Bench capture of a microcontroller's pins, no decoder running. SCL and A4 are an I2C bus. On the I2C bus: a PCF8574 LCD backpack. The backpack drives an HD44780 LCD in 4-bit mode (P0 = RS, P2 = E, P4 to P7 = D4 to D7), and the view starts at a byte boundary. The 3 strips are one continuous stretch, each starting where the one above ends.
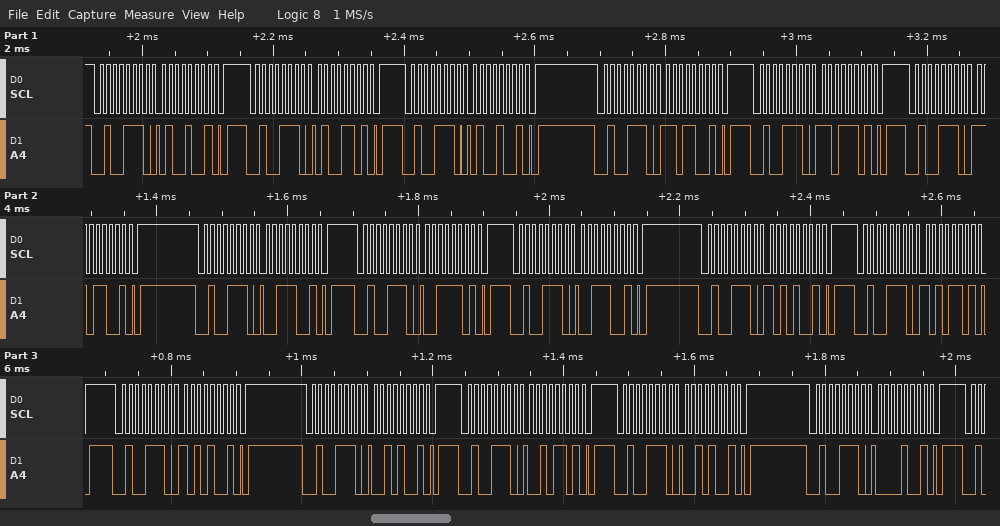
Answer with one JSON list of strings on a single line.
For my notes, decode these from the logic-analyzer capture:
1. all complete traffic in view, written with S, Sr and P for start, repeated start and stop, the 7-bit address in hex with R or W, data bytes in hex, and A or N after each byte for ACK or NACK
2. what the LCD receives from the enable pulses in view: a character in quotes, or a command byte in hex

["S 27W A 49 A P S 27W A 4D A P S 27W A 49 A P S 27W A D9 A P S 27W A DD A P S 27W A D9 A P S 27W A 39 A P S 27W A 3D A P S 27W A 39 A P S 27W A A9 A P S 27W A AD A P S 27W A A9 A P S 27W A 29 A P S 27W A 2D A P S 27W A 29 A P S 27W A 09 A P", "'M' ':'"]
